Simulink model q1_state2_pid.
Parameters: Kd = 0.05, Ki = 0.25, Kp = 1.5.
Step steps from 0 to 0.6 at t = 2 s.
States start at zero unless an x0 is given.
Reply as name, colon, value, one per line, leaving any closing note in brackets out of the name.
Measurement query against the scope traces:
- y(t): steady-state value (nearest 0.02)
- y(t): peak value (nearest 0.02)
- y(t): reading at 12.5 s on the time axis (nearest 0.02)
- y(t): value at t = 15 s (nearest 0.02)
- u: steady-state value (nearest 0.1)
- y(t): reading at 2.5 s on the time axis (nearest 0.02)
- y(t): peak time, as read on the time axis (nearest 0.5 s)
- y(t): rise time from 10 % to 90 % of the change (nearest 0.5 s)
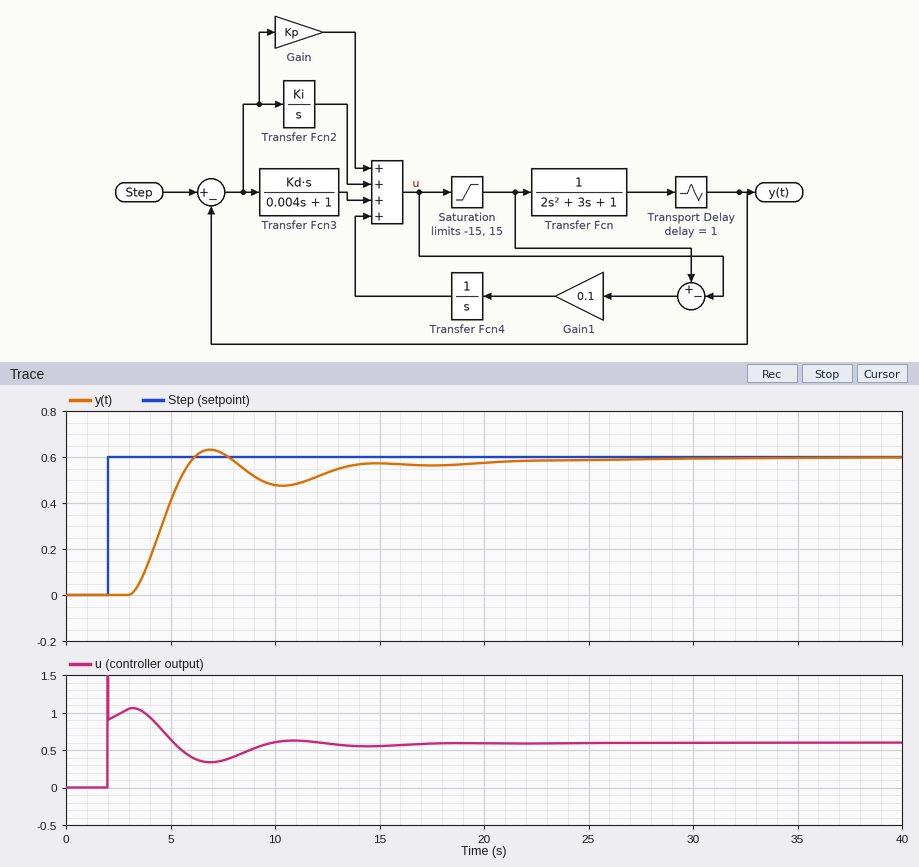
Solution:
y(t): steady-state value: 0.60
y(t): peak value: 0.64
y(t): reading at 12.5 s on the time axis: 0.54
y(t): value at t = 15 s: 0.58
u: steady-state value: 0.6
y(t): reading at 2.5 s on the time axis: 0.00
y(t): peak time, as read on the time axis: 7.0 s
y(t): rise time from 10 % to 90 % of the change: 2.0 s
